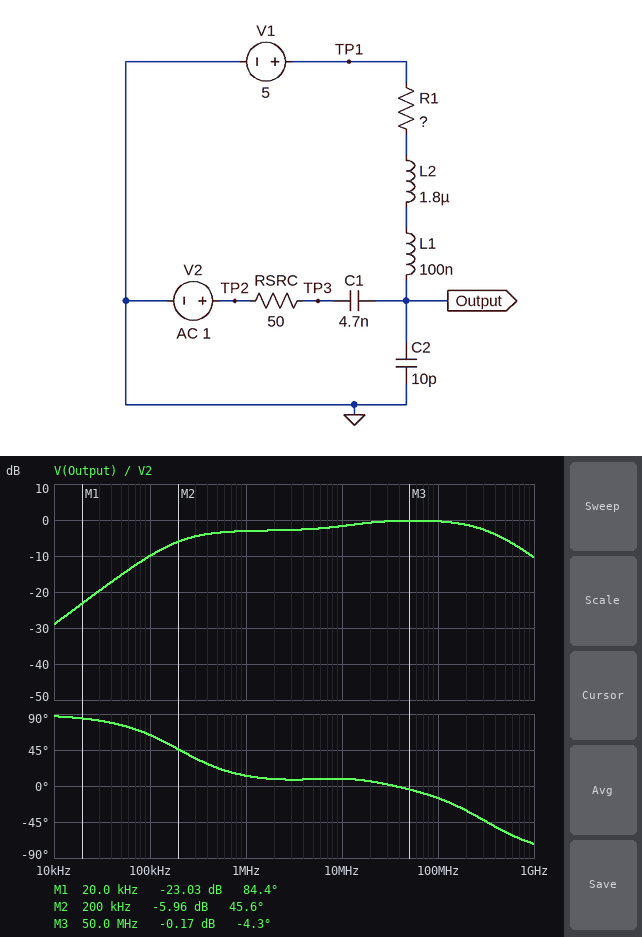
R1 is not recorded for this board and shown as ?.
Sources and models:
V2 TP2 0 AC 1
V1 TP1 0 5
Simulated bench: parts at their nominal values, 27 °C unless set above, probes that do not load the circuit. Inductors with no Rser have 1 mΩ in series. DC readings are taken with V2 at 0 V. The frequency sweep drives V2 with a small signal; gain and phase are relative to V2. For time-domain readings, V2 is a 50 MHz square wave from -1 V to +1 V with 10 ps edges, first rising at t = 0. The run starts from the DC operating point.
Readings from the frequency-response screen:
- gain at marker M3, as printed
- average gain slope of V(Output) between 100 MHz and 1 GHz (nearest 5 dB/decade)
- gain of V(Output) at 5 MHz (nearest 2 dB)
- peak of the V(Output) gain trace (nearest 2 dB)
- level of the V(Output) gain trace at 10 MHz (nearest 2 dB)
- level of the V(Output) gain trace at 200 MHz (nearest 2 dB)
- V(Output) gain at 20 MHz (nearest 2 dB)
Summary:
-0.17 dB
-10 dB/decade
-2 dB
0 dB
-2 dB
-2 dB
0 dB
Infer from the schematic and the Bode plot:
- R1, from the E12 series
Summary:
120 Ω
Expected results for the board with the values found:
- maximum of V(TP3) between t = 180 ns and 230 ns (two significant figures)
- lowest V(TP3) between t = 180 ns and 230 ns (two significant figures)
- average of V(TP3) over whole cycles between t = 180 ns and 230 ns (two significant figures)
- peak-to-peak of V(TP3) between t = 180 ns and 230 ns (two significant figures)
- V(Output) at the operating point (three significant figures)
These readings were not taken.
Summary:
830 mV
-1.3 V
-230 mV
2.1 V
5.00 V
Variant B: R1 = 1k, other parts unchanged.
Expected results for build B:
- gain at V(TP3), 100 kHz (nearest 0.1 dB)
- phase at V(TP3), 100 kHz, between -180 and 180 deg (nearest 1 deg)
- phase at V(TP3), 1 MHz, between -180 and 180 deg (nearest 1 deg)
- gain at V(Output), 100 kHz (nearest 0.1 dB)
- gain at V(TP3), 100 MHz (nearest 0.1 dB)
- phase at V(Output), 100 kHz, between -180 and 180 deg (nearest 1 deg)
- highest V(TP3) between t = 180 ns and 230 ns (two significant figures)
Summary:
-0.4 dB
-1 deg
0 deg
-0.9 dB
-0.5 dB
18 deg
940 mV
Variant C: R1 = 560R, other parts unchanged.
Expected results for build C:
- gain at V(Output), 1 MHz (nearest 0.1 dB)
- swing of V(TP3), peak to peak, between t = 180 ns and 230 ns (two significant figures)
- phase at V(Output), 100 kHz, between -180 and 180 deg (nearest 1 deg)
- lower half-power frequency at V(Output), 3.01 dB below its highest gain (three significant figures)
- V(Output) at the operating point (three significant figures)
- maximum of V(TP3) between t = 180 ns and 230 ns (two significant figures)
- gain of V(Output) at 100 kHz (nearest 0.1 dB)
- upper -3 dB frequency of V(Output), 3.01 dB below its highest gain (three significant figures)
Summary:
-0.8 dB
2.0 V
29 deg
60.6 kHz
5.00 V
930 mV
-1.9 dB
349 MHz
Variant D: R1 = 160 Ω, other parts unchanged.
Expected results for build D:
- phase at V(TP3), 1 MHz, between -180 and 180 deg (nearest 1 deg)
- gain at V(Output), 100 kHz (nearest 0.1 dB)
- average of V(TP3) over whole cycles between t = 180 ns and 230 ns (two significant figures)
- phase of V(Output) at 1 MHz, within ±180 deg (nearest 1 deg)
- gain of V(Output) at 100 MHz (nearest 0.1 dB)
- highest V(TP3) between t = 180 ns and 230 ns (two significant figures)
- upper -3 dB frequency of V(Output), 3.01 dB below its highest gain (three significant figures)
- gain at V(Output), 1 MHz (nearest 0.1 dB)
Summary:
-2 deg
-7.9 dB
-200 mV
10 deg
-0.4 dB
860 mV
336 MHz
-2.4 dB
